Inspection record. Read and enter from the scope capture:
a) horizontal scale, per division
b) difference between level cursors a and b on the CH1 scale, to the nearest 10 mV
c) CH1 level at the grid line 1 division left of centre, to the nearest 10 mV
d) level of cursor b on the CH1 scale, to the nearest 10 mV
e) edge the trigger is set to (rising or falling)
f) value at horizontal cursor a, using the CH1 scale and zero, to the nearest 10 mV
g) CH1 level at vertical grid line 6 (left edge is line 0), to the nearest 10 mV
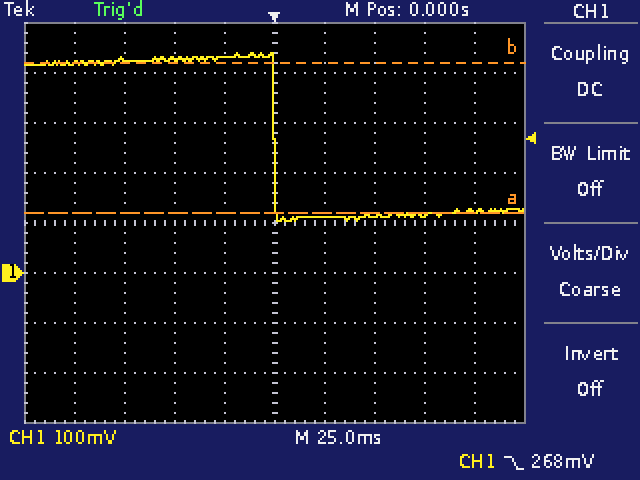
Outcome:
25 ms
300 mV
430 mV
420 mV
falling
120 mV
110 mV
